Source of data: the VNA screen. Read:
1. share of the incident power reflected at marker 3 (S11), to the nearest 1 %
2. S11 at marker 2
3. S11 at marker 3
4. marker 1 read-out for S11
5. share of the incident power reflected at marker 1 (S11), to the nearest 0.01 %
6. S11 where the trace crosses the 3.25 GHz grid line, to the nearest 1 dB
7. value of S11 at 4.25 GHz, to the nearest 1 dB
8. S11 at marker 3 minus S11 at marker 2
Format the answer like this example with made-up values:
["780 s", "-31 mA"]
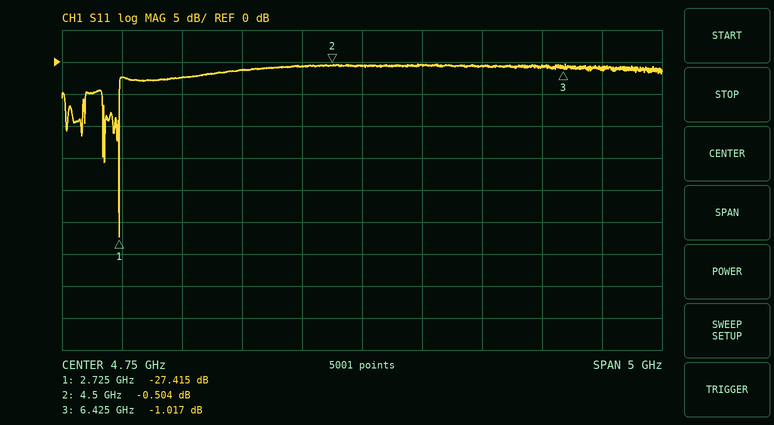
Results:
["79 %", "-0.504 dB", "-1.017 dB", "-27.415 dB", "0.18 %", "-2 dB", "-1 dB", "-0.513 dB"]
